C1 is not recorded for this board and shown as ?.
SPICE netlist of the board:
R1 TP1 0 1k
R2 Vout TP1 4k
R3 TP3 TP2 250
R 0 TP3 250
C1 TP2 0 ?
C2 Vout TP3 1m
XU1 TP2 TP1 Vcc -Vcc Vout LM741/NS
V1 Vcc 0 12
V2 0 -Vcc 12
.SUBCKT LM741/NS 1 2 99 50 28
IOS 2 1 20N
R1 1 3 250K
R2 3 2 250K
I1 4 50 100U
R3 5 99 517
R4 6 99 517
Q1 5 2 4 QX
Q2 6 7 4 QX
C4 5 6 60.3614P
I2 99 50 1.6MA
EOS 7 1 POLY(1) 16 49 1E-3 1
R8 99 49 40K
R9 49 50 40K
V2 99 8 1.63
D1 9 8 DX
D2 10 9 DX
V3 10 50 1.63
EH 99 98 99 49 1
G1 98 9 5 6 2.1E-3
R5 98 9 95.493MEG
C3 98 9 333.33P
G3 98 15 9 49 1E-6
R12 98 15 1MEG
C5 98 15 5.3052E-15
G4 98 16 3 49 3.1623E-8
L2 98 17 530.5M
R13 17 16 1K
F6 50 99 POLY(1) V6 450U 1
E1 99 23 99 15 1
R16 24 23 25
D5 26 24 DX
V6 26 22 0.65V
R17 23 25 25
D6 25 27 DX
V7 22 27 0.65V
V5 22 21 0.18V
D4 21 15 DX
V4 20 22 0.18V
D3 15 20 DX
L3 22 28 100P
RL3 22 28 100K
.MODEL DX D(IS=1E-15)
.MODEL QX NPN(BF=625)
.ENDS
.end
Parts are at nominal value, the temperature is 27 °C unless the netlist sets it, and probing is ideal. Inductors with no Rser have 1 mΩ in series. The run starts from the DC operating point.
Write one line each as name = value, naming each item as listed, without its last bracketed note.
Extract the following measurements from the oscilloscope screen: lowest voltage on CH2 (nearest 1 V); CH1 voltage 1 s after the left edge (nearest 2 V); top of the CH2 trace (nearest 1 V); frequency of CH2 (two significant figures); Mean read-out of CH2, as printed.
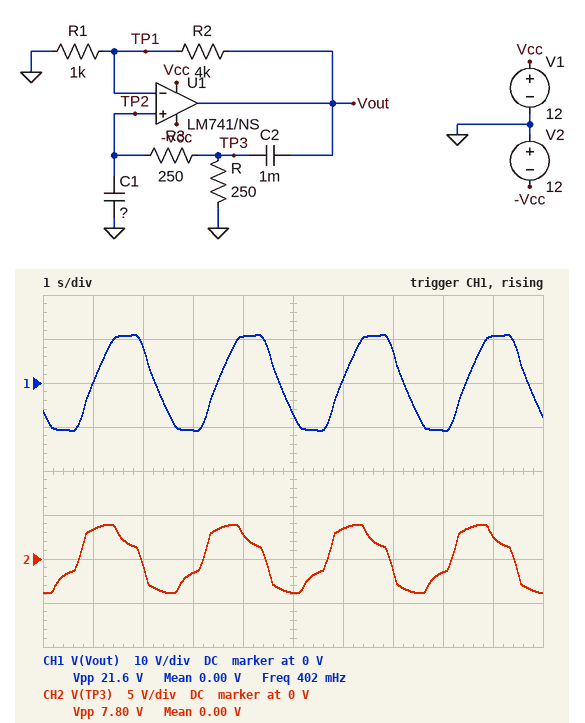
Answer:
lowest voltage on CH2 = -4 V
CH1 voltage 1 s after the left edge = 0 V
top of the CH2 trace = 4 V
frequency of CH2 = 400 mHz
Mean read-out of CH2, as printed = 0.00 V
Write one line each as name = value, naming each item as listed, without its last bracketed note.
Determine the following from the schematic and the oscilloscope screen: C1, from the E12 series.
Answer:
C1, from the E12 series = 1.5 mF
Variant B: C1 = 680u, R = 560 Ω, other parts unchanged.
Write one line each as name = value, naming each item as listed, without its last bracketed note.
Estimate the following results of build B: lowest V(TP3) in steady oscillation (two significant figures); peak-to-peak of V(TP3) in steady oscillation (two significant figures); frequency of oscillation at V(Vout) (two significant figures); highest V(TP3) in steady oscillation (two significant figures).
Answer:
lowest V(TP3) in steady oscillation = -8.0 V
peak-to-peak of V(TP3) in steady oscillation = 16 V
frequency of oscillation at V(Vout) = 250 mHz
highest V(TP3) in steady oscillation = 8.0 V
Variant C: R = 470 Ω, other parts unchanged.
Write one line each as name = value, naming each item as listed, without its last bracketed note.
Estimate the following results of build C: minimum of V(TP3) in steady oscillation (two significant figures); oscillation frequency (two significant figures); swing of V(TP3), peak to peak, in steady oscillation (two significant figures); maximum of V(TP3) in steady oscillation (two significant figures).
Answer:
minimum of V(TP3) in steady oscillation = -5.6 V
oscillation frequency = 260 mHz
swing of V(TP3), peak to peak, in steady oscillation = 11 V
maximum of V(TP3) in steady oscillation = 5.6 V
